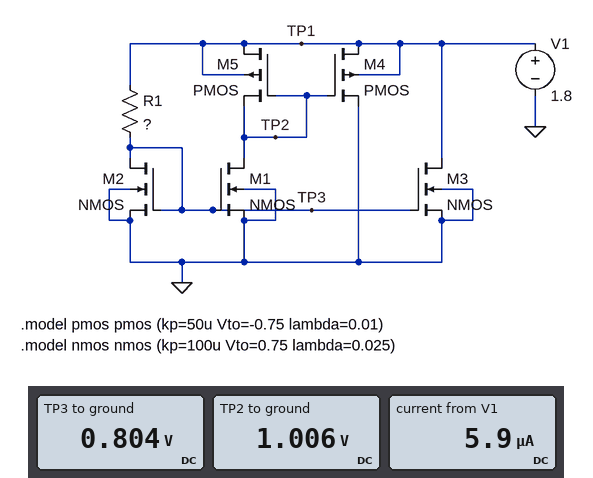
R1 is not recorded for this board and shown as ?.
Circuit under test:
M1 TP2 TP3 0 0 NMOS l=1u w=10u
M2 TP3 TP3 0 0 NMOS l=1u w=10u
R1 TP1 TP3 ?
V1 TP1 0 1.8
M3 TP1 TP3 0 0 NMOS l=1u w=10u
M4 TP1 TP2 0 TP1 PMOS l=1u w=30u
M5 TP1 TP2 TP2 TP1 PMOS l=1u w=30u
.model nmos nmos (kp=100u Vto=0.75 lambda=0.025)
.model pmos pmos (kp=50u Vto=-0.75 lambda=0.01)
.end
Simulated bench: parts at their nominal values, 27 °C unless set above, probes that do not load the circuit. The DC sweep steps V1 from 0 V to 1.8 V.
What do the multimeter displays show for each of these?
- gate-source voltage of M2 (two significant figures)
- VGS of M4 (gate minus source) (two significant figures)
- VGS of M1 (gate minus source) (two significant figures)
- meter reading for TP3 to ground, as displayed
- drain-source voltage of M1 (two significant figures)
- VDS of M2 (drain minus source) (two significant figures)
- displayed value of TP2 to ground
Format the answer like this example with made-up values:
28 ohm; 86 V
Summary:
800 mV; 1.0 V; 800 mV; 0.804 V; 1.0 V; 800 mV; 1.006 V
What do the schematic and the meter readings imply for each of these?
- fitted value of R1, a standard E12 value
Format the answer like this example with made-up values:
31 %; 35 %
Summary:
680 kΩ
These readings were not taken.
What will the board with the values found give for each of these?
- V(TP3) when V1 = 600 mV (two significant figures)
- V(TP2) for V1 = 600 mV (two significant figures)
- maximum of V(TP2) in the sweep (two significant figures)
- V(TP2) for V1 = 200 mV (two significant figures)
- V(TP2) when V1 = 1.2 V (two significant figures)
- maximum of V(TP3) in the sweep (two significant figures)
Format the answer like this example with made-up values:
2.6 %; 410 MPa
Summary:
600 mV; 300 mV; 1.0 V; 100 mV; 420 mV; 800 mV
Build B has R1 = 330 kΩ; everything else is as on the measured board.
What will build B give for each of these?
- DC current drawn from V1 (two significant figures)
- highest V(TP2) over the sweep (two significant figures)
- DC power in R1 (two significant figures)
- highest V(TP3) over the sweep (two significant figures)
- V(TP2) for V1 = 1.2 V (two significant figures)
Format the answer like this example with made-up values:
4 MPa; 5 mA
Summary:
12 µA; 990 mV; 2.9 µW; 830 mV; 410 mV
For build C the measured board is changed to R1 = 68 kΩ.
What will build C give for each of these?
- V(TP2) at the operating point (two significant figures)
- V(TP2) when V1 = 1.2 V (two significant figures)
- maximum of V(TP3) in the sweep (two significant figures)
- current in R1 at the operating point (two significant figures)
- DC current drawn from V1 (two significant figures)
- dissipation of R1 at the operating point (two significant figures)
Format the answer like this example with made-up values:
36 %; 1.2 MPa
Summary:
920 mV; 370 mV; 910 mV; 13 µA; 53 µA; 12 µW
